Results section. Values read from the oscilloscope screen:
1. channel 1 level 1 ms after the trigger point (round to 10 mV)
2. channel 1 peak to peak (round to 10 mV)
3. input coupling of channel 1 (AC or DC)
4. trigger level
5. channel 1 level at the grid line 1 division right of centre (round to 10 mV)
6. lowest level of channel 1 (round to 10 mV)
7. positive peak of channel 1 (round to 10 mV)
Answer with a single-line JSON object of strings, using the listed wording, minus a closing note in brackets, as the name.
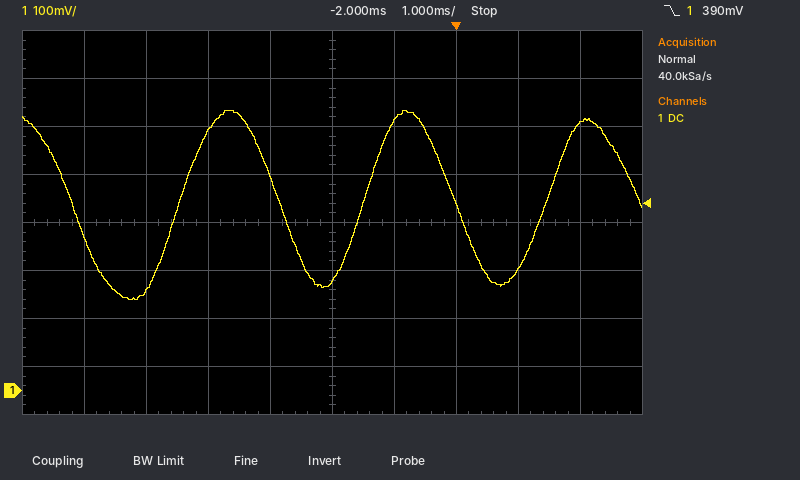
{"channel 1 level 1 ms after the trigger point": "250 mV", "channel 1 peak to peak": "390 mV", "input coupling of channel 1": "DC", "trigger level": "390 mV", "channel 1 level at the grid line 1 division right of centre": "560 mV", "lowest level of channel 1": "190 mV", "positive peak of channel 1": "580 mV"}
